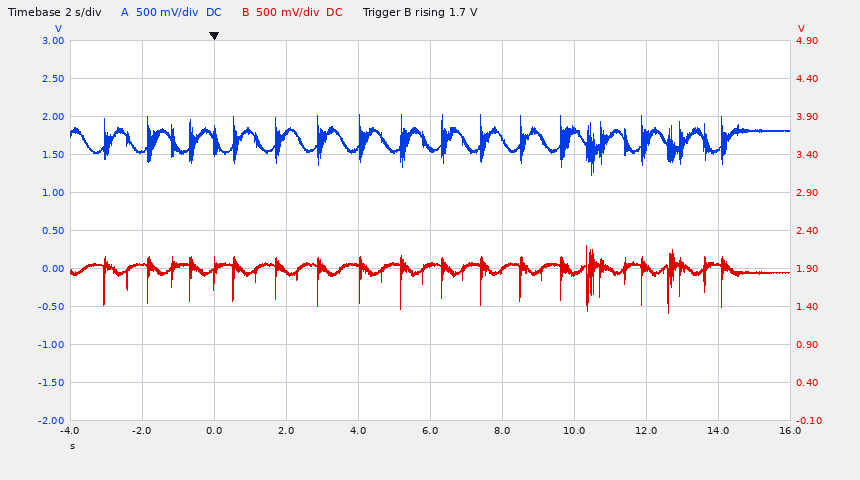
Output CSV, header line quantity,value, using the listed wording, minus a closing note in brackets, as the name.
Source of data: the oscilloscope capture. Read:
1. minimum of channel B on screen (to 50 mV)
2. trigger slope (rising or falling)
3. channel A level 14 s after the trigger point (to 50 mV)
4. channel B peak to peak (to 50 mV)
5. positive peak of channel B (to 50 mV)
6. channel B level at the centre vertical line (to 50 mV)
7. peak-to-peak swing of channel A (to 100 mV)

quantity,value
minimum of channel B on screen,1.30 V
trigger slope,rising
channel A level 14 s after the trigger point,1.55 V
channel B peak to peak,900 mV
positive peak of channel B,2.20 V
channel B level at the centre vertical line,1.95 V
peak-to-peak swing of channel A,800 mV
